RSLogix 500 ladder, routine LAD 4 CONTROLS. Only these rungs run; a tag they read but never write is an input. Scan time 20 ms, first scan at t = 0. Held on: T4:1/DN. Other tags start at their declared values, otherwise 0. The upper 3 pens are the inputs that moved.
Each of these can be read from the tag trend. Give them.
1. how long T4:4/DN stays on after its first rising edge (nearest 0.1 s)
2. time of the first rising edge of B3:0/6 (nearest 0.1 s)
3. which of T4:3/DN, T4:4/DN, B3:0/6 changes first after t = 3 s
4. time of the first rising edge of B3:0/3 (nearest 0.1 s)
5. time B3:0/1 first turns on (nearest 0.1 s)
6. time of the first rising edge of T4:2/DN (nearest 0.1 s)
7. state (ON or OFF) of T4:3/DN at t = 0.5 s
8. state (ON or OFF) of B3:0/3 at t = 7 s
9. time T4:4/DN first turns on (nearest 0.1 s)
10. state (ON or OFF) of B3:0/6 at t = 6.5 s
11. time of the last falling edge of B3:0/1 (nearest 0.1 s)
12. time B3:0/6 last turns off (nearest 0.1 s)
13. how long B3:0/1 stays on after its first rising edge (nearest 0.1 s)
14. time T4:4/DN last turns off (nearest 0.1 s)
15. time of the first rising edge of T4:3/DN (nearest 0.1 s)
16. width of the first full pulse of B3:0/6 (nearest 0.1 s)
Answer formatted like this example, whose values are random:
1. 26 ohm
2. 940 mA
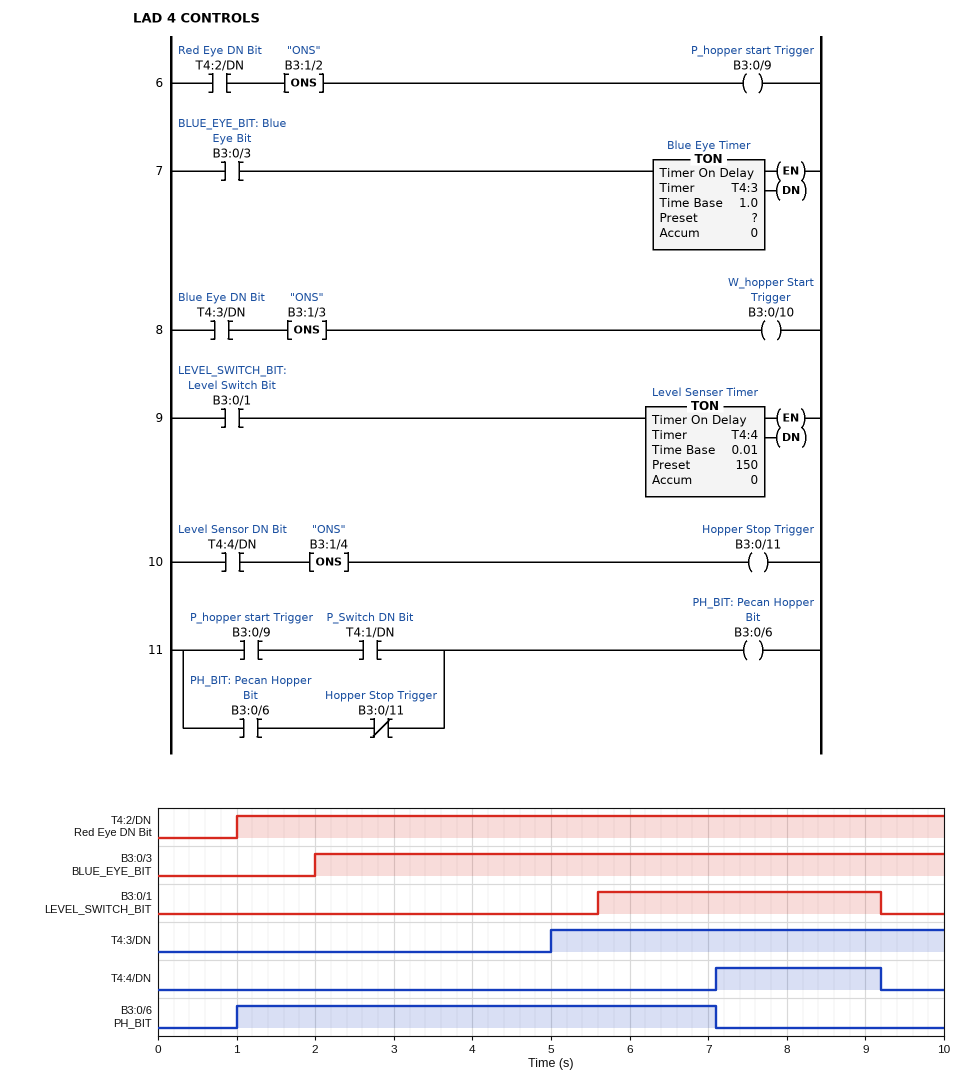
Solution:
1. 2.1 s
2. 1.0 s
3. T4:3/DN
4. 2.0 s
5. 5.6 s
6. 1.0 s
7. OFF
8. ON
9. 7.1 s
10. ON
11. 9.2 s
12. 7.1 s
13. 3.6 s
14. 9.2 s
15. 5.0 s
16. 6.1 s
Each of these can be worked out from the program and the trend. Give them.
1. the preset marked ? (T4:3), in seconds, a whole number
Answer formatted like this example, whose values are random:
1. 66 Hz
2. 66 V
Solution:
1. 3 s
